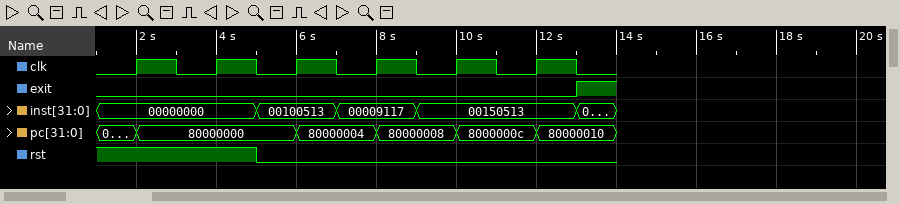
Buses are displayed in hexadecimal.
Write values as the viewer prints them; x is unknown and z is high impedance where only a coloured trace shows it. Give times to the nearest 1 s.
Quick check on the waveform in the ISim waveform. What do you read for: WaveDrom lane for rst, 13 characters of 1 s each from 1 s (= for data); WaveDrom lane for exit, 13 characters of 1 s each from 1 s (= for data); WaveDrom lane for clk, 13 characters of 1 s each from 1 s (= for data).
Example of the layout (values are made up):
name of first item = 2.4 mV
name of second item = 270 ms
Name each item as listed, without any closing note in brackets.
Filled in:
WaveDrom lane for rst, 13 characters of 1 s each from 1 s = {name: 'rst', wave: '1...0........'}
WaveDrom lane for exit, 13 characters of 1 s each from 1 s = {name: 'exit', wave: '0...........1'}
WaveDrom lane for clk, 13 characters of 1 s each from 1 s = {name: 'clk', wave: '0101010101010'}
